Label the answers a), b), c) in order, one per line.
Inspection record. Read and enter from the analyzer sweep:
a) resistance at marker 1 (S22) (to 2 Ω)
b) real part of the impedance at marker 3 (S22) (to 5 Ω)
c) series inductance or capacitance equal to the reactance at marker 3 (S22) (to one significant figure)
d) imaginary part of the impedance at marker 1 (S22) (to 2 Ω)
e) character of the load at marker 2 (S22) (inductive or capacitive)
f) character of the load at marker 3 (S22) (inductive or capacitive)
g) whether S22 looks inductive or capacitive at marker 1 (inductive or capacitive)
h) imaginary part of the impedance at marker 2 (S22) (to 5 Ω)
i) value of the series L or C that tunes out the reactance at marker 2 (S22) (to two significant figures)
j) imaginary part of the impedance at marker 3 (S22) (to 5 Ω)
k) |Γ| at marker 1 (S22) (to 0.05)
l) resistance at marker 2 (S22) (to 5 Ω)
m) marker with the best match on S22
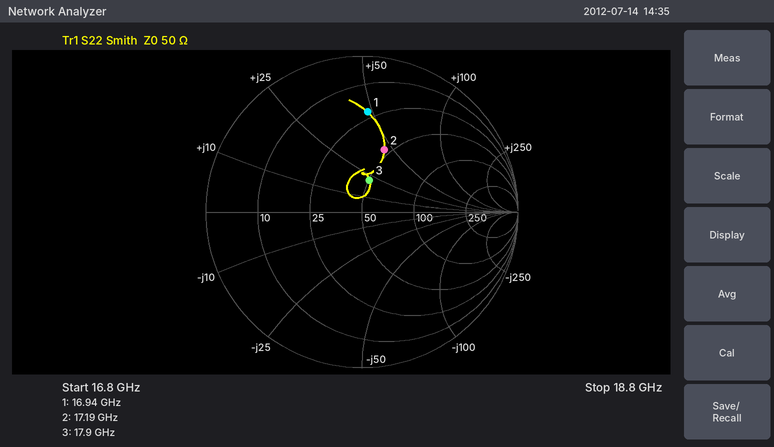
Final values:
a) 22 Ω
b) 50 Ω
c) 200 pH
d) +48 Ω
e) inductive
f) inductive
g) inductive
h) +45 Ω
i) 210 fF
j) +20 Ω
k) 0.65
l) 45 Ω
m) marker 3
